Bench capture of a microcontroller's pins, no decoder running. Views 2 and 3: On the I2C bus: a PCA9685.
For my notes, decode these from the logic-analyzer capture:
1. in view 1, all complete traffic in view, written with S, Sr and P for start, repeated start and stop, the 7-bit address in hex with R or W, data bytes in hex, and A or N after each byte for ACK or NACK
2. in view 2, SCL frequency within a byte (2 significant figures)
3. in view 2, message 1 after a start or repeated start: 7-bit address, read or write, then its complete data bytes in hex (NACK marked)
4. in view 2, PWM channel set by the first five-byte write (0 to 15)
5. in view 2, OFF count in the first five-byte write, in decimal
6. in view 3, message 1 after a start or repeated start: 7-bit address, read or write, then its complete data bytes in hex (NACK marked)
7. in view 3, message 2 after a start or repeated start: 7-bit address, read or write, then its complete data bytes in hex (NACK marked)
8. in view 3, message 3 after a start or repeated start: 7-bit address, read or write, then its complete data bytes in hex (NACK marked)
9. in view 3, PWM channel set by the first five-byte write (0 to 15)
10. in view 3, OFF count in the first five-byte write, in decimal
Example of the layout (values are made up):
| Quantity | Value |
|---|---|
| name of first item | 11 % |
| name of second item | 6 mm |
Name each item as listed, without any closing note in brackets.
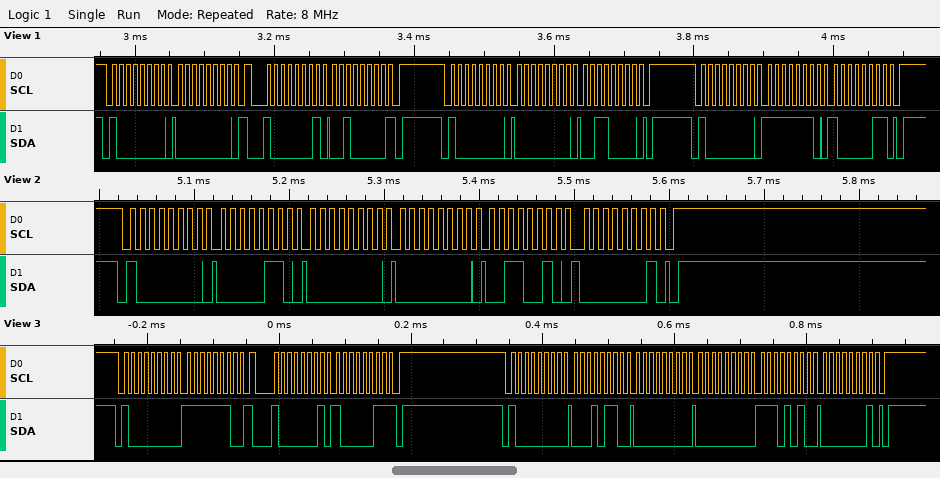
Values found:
| Quantity | Value |
|---|---|
| in view 1, all complete traffic in view, written with S, Sr and P for start, repeated start and stop, the 7-bit address in hex with R or W, data bytes in hex, and A or N after each byte for ACK or NACK | S 40W A 00 A Sr 40R A 20 N P S 40W A 00 A 30 A P S 40W A FE A 83 A P |
| in view 2, SCL frequency within a byte | 100 kHz |
| in view 2, message 1 after a start or repeated start: 7-bit address, read or write, then its complete data bytes in hex | 0x40 write: 06 00 00 32 01 |
| in view 2, PWM channel set by the first five-byte write | 0 |
| in view 2, OFF count in the first five-byte write, in decimal | 306 |
| in view 3, message 1 after a start or repeated start: 7-bit address, read or write, then its complete data bytes in hex | 0x40 write: FE |
| in view 3, message 2 after a start or repeated start: 7-bit address, read or write, then its complete data bytes in hex | 0x40 read: 83 NACK |
| in view 3, message 3 after a start or repeated start: 7-bit address, read or write, then its complete data bytes in hex | 0x40 write: 16 00 00 EA 01 |
| in view 3, PWM channel set by the first five-byte write | 4 |
| in view 3, OFF count in the first five-byte write, in decimal | 490 |
